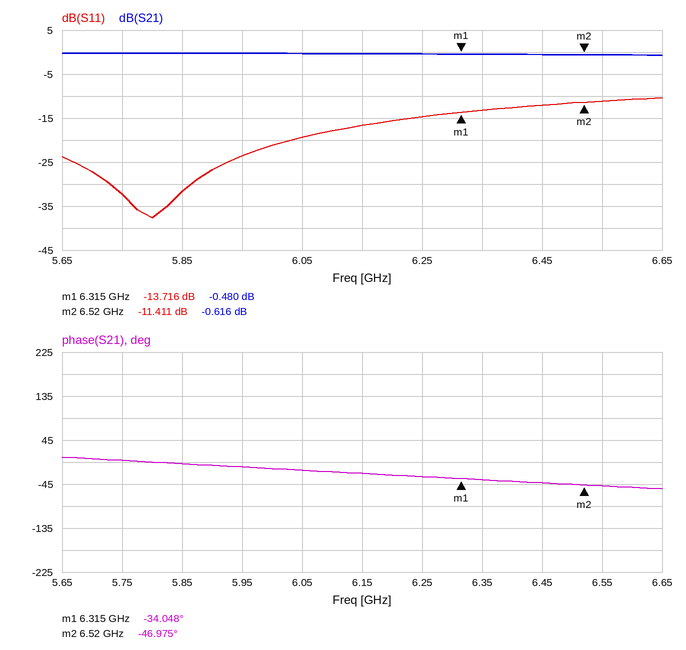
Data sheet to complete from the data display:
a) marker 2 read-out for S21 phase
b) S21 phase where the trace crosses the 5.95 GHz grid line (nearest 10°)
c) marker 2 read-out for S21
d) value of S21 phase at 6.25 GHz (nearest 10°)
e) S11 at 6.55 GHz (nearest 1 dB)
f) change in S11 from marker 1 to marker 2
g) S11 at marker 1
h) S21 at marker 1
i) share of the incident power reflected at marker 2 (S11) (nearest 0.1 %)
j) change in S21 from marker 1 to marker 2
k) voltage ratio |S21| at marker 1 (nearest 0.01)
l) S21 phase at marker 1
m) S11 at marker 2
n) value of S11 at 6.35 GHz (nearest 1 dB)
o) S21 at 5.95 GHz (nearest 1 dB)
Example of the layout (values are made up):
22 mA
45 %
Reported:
-46.975°
-10°
-0.616 dB
-30°
-11 dB
2.305 dB
-13.716 dB
-0.480 dB
7.2 %
-0.136 dB
0.95
-34.048°
-11.411 dB
-13 dB
0 dB
